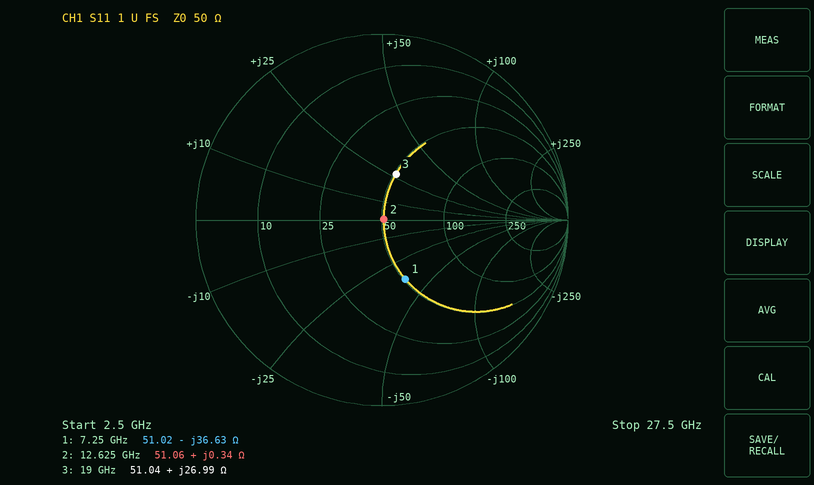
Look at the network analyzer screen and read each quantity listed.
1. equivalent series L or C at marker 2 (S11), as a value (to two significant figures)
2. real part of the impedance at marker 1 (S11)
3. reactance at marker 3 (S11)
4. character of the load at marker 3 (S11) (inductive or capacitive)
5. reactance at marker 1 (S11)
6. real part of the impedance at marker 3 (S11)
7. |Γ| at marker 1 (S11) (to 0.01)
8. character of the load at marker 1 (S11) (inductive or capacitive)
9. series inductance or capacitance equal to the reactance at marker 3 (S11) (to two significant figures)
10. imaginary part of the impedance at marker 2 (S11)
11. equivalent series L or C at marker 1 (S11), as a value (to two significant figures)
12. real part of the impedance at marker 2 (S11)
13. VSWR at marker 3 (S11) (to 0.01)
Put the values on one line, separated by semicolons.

4.3 pH; 51.02 Ω; +26.99 Ω; inductive; -36.63 Ω; 51.04 Ω; 0.34; capacitive; 230 pH; +0.34 Ω; 600 fF; 51.06 Ω; 1.70
